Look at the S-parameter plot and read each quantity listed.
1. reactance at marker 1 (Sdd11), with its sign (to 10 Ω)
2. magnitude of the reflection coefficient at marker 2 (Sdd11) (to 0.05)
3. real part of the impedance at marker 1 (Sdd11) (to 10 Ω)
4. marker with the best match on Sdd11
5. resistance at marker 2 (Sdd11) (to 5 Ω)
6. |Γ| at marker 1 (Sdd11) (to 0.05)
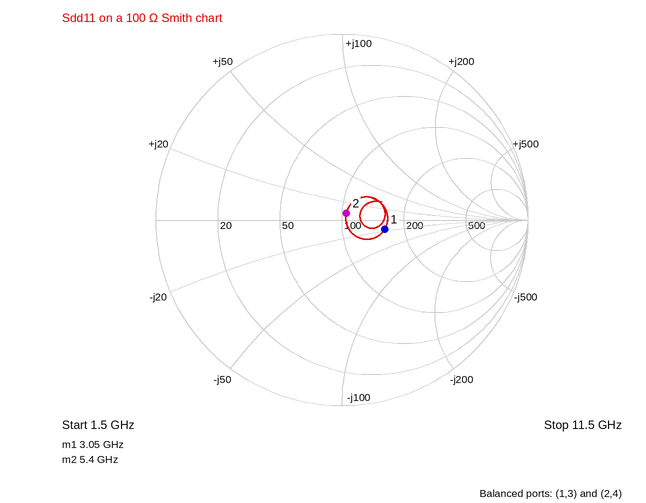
-20 Ω
0.05
160 Ω
marker 2
105 Ω
0.25
